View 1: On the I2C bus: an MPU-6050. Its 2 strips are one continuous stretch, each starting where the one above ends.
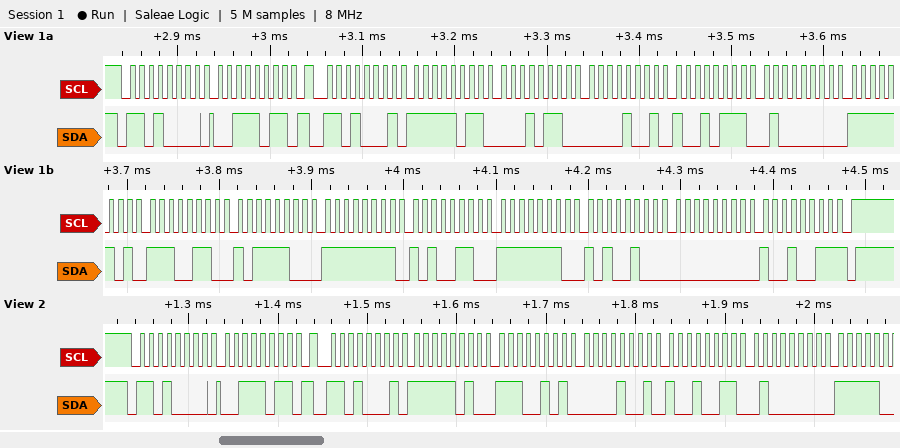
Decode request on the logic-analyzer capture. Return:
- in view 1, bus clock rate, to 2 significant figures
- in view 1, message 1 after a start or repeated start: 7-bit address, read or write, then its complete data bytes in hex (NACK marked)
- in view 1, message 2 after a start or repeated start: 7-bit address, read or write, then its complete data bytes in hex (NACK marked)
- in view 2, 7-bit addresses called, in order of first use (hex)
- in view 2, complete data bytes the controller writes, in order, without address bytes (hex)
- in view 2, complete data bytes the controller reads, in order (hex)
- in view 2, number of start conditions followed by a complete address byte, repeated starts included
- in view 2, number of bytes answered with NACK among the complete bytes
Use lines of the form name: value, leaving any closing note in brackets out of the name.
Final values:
in view 1, bus clock rate, to 2 significant figures: 100 kHz
in view 1, message 1 after a start or repeated start: 7-bit address, read or write, then its complete data bytes in hex: 0x68 write: 3B
in view 1, message 2 after a start or repeated start: 7-bit address, read or write, then its complete data bytes in hex: 0x68 read: FB 16 09 97 40 FD E6 BC FF A6 FE A4 00 93 NACK
in view 2, 7-bit addresses called, in order of first use: 0x68
in view 2, complete data bytes the controller writes, in order, without address bytes: 3B
in view 2, complete data bytes the controller reads, in order: FA E5 09 93 40
in view 2, number of start conditions followed by a complete address byte, repeated starts included: 2
in view 2, number of bytes answered with NACK among the complete bytes: 0
